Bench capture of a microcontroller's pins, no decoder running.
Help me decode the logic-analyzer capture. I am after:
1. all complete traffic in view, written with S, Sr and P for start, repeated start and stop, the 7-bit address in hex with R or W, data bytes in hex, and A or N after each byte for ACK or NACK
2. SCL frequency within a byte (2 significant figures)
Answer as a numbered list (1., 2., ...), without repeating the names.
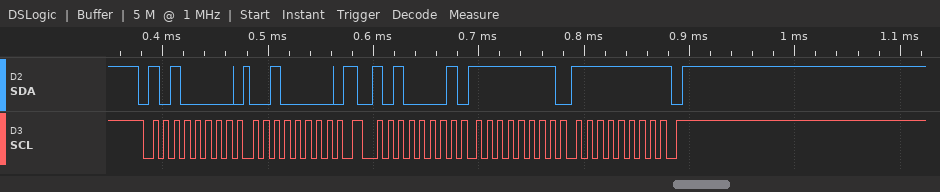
1. S 50W A 20 A Sr 50R A FF A FF N P
2. 100 kHz
